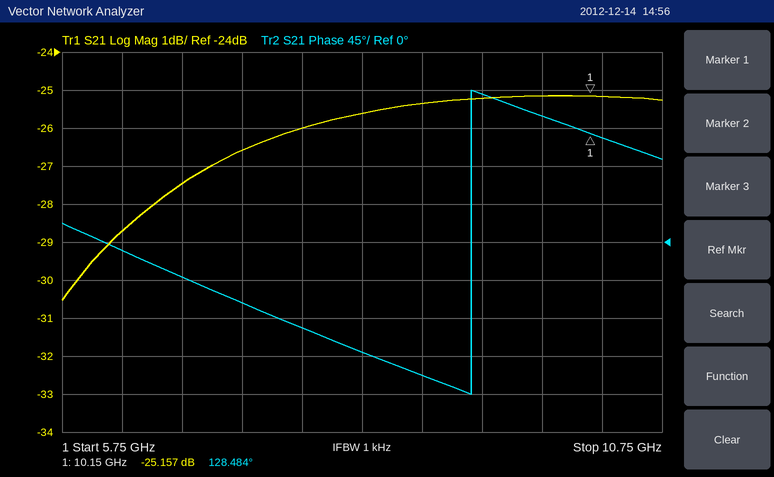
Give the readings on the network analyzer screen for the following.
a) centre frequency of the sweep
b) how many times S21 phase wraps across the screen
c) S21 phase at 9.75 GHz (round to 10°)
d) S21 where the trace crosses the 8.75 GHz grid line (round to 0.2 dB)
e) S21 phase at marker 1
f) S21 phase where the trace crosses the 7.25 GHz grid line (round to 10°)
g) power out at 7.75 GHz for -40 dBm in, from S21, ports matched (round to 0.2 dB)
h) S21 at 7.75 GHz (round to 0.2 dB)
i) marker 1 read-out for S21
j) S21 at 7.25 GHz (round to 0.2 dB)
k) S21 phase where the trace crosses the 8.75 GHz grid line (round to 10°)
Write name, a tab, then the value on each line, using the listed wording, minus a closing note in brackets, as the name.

centre frequency of the sweep	8.25 GHz
how many times S21 phase wraps across the screen	1
S21 phase at 9.75 GHz	150°
S21 where the trace crosses the 8.75 GHz grid line	-25.4 dB
S21 phase at marker 1	128.484°
S21 phase where the trace crosses the 7.25 GHz grid line	-70°
power out at 7.75 GHz for -40 dBm in, from S21, ports matched	-66.0 dBm
S21 at 7.75 GHz	-26.0 dB
marker 1 read-out for S21	-25.157 dB
S21 at 7.25 GHz	-26.6 dB
S21 phase where the trace crosses the 8.75 GHz grid line	-160°
